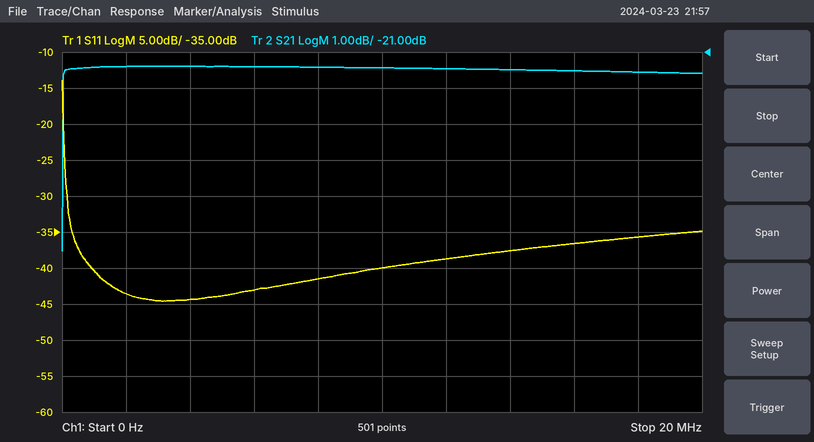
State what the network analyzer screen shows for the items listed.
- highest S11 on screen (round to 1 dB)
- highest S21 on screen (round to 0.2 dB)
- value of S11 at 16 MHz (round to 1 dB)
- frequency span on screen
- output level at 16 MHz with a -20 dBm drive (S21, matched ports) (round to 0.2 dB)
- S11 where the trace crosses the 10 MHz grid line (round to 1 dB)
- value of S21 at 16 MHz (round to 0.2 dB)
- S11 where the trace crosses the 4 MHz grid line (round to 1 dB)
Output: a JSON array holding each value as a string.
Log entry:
["-14 dB", "-21.4 dB", "-37 dB", "20 MHz", "-41.6 dBm", "-40 dB", "-21.6 dB", "-44 dB"]
